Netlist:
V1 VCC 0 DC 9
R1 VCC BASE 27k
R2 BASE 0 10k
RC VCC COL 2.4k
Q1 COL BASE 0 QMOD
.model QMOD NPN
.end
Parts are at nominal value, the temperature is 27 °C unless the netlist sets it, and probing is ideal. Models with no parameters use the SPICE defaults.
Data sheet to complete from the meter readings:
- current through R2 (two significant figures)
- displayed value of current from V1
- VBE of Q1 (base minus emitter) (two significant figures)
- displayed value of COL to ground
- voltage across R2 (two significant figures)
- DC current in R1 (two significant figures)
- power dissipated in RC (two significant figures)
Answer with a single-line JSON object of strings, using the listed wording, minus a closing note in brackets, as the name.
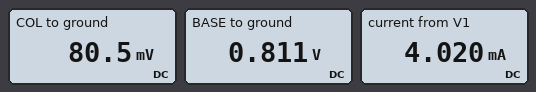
{"current through R2": "81 µA", "displayed value of current from V1": "4.020 mA", "VBE of Q1 (base minus emitter)": "810 mV", "displayed value of COL to ground": "80.5 mV", "voltage across R2": "810 mV", "DC current in R1": "300 µA", "power dissipated in RC": "33 mW"}
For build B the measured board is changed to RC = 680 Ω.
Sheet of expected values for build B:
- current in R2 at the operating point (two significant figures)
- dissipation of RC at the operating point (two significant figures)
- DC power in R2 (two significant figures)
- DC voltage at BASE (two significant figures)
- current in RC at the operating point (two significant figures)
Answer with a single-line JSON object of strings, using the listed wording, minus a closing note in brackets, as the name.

{"current in R2 at the operating point": "84 µA", "dissipation of RC at the operating point": "120 mW", "DC power in R2": "71 µW", "DC voltage at BASE": "840 mV", "current in RC at the operating point": "13 mA"}
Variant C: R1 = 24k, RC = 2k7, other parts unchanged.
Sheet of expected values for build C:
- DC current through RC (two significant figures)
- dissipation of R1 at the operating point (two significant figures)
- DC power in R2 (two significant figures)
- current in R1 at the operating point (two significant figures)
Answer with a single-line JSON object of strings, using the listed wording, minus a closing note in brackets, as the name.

{"DC current through RC": "3.3 mA", "dissipation of R1 at the operating point": "2.8 mW", "DC power in R2": "65 µW", "current in R1 at the operating point": "340 µA"}
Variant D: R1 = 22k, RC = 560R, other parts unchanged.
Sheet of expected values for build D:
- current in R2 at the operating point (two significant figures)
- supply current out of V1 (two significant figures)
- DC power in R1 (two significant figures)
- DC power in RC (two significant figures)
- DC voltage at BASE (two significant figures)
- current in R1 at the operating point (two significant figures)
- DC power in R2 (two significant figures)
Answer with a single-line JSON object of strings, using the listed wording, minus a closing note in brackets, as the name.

{"current in R2 at the operating point": "85 µA", "supply current out of V1": "16 mA", "DC power in R1": "3.0 mW", "DC power in RC": "140 mW", "DC voltage at BASE": "850 mV", "current in R1 at the operating point": "370 µA", "DC power in R2": "72 µW"}
